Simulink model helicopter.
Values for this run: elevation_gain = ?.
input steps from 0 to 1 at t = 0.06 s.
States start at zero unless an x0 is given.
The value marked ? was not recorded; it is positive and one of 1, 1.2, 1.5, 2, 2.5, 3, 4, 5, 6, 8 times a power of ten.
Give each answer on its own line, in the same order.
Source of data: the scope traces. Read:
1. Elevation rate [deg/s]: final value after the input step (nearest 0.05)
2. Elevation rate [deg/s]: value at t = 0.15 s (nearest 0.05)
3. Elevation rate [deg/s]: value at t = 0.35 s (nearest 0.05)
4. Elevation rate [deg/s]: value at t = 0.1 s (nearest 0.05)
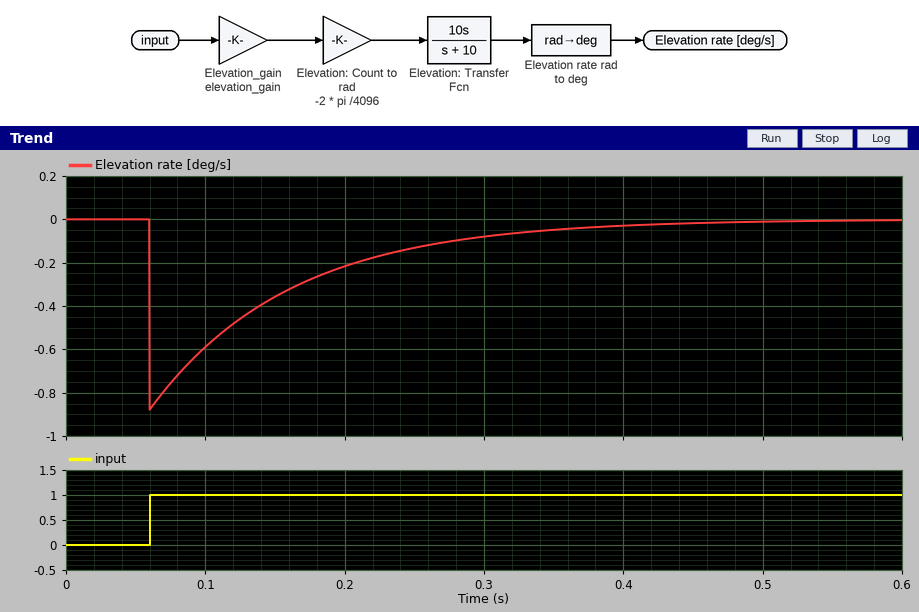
0.00
-0.35
-0.05
-0.60
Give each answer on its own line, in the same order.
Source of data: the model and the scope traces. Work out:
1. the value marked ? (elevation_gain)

1
